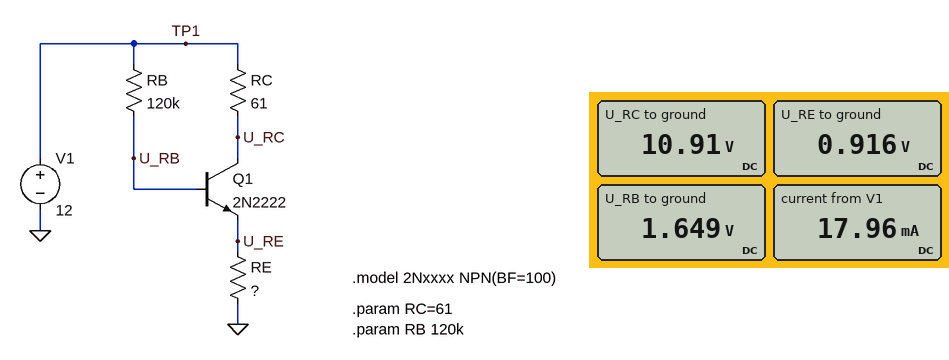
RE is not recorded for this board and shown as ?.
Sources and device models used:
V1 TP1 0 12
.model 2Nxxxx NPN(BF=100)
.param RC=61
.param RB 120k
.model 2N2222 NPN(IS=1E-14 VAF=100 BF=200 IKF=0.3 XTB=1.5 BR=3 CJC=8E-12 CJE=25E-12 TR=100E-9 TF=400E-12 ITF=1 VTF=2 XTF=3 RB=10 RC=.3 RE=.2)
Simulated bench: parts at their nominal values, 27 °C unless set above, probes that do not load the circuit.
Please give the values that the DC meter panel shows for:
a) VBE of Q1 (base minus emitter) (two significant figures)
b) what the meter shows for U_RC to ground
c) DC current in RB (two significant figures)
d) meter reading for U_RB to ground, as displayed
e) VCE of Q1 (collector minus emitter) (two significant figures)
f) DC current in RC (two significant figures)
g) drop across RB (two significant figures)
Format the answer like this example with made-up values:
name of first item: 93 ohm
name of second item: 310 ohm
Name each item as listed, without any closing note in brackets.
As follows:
VBE of Q1 (base minus emitter): 730 mV
what the meter shows for U_RC to ground: 10.91 V
DC current in RB: 86 µA
meter reading for U_RB to ground, as displayed: 1.649 V
VCE of Q1 (collector minus emitter): 10 V
DC current in RC: 18 mA
drop across RB: 10 V
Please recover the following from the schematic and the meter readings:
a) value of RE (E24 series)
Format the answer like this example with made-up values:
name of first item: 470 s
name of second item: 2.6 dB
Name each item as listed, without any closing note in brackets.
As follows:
value of RE: 51 Ω
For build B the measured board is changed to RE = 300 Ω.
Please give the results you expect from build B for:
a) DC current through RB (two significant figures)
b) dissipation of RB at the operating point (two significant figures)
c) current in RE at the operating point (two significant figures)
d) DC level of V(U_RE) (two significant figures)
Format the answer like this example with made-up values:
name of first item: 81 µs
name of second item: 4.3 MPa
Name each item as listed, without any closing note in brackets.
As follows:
DC current through RB: 62 µA
dissipation of RB at the operating point: 460 µW
current in RE at the operating point: 13 mA
DC level of V(U_RE): 3.8 V
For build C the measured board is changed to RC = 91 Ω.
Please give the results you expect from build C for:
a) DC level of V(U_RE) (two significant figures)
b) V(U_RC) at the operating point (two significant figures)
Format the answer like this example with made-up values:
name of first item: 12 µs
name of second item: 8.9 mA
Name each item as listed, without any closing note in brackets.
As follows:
DC level of V(U_RE): 910 mV
V(U_RC) at the operating point: 10 V
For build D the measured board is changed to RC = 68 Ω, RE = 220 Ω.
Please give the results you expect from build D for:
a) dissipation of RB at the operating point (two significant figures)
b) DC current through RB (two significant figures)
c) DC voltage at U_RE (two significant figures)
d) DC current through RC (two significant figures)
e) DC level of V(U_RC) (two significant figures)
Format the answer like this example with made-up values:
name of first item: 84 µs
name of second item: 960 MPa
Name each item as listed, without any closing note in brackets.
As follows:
dissipation of RB at the operating point: 560 µW
DC current through RB: 68 µA
DC voltage at U_RE: 3.1 V
DC current through RC: 14 mA
DC level of V(U_RC): 11 V
